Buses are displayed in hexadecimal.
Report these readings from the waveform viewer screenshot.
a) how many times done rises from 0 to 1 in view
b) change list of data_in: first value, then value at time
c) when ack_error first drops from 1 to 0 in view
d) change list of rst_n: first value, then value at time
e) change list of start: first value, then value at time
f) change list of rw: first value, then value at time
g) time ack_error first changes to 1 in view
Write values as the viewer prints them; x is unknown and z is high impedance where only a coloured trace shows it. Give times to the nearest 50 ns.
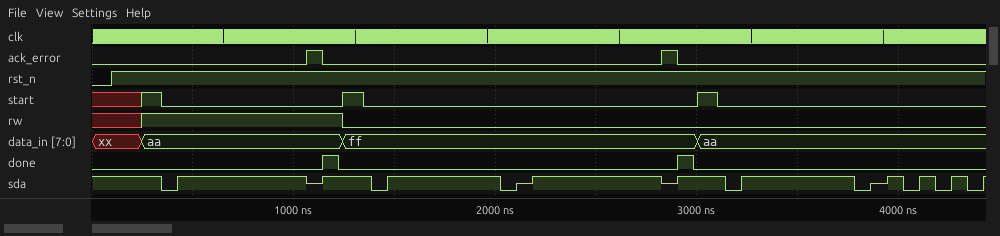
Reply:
2
xx, aa at 250 ns, ff at 1250 ns, aa at 3000 ns
1150 ns
0, 1 at 100 ns
x, 1 at 250 ns, 0 at 350 ns, 1 at 1250 ns, 0 at 1350 ns, 1 at 3000 ns, 0 at 3100 ns
x, 1 at 250 ns, 0 at 1250 ns
1050 ns
